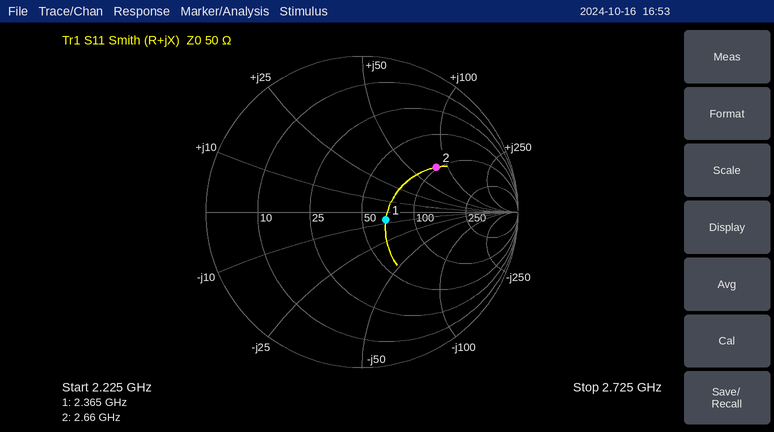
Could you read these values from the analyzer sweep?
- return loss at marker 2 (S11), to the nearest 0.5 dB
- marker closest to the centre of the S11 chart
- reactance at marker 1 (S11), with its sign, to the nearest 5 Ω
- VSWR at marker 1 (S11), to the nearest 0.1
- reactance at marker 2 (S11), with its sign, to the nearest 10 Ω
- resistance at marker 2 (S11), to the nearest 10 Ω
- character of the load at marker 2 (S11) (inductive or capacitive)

5.0 dB
marker 1
-5 Ω
1.4
+80 Ω
100 Ω
inductive
